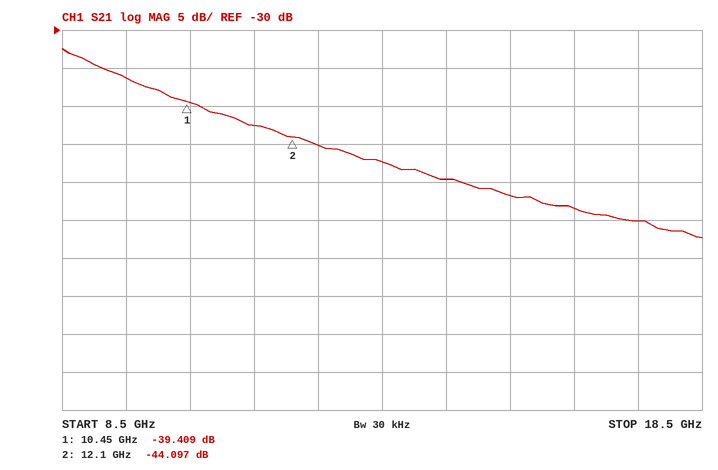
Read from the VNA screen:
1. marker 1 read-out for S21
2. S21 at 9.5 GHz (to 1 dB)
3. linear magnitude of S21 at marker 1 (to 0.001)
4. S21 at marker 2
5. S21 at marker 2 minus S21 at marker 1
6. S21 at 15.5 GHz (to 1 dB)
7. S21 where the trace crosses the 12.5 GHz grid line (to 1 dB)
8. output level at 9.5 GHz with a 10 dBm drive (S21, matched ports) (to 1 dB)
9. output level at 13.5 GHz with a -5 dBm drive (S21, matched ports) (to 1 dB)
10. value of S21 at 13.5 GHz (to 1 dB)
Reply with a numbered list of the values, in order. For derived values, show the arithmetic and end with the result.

1. -39.409 dB
2. -36 dB
3. 10^(-39.409/20) ≈ 0.011
4. -44.097 dB
5. -44.097 − (-39.409) = -4.688 dB
6. -52 dB
7. -45 dB
8. 10 dBm + (-36 dB) = -26 dBm
9. -5 dBm + (-47 dB) = -52 dBm
10. -47 dB
